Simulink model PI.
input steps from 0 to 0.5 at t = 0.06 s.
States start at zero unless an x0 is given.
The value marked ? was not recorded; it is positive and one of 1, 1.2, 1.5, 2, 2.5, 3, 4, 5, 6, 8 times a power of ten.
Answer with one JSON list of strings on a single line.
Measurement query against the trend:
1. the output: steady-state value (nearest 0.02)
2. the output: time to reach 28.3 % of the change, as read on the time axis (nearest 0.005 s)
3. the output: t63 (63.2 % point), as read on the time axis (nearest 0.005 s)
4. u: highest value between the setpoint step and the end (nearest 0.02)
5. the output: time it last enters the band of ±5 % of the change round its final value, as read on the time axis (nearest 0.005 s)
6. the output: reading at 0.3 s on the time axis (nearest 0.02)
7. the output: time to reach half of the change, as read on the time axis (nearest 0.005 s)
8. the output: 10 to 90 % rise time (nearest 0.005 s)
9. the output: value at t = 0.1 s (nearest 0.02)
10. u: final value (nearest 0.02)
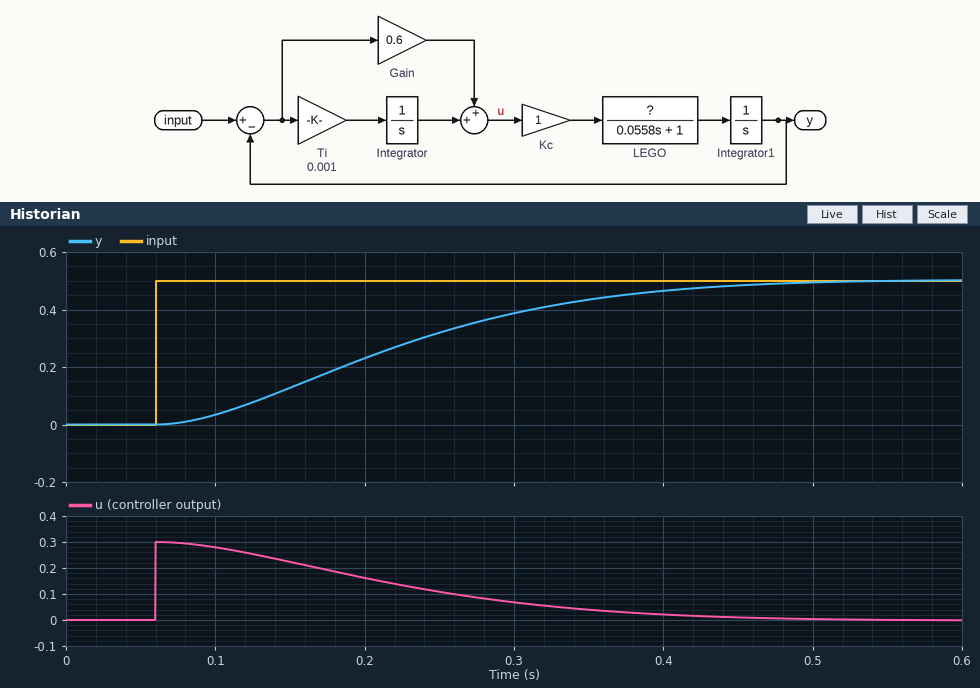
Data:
["0.50", "0.155 s", "0.250 s", "0.30", "0.425 s", "0.38", "0.210 s", "0.265 s", "0.04", "0.00"]
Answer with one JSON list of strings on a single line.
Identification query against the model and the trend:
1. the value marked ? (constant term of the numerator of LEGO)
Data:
["10"]
